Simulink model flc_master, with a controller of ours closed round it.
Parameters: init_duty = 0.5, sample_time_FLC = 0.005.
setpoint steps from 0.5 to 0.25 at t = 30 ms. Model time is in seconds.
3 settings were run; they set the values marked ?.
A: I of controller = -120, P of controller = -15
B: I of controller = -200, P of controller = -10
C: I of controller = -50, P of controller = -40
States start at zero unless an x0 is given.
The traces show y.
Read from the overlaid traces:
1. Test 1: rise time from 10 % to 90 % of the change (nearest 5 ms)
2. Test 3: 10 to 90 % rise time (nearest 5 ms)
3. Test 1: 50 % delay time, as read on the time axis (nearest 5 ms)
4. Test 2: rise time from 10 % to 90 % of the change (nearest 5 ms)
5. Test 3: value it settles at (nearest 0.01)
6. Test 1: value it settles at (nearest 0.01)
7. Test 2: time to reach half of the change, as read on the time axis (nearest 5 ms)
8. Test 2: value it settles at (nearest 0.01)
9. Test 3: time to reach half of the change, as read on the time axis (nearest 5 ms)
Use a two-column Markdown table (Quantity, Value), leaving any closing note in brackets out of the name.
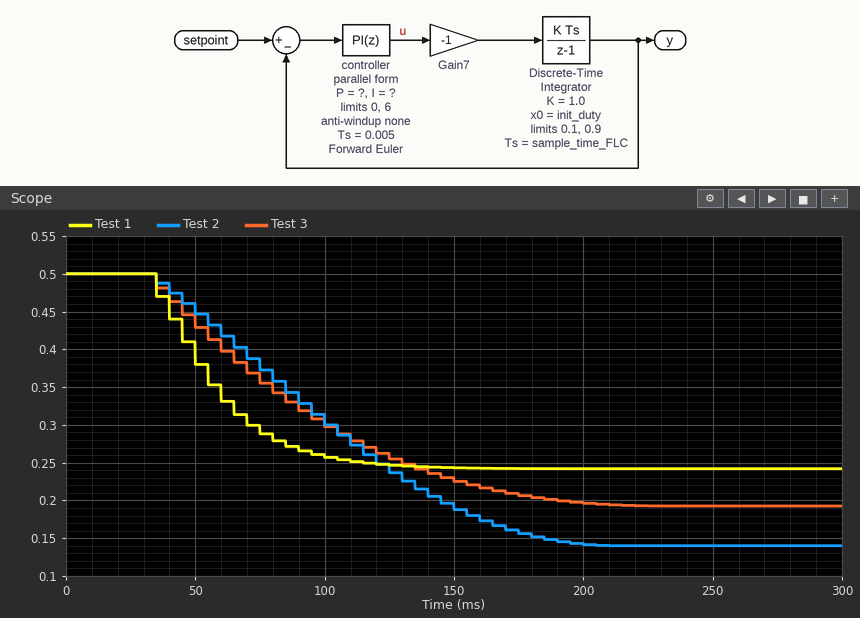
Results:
| Quantity | Value |
|---|---|
| Test 1: rise time from 10 % to 90 % of the change | 55 ms |
| Test 3: 10 to 90 % rise time | 115 ms |
| Test 1: 50 % delay time, as read on the time axis | 55 ms |
| Test 2: rise time from 10 % to 90 % of the change | 115 ms |
| Test 3: value it settles at | 0.19 |
| Test 1: value it settles at | 0.24 |
| Test 2: time to reach half of the change, as read on the time axis | 95 ms |
| Test 2: value it settles at | 0.14 |
| Test 3: time to reach half of the change, as read on the time axis | 80 ms |
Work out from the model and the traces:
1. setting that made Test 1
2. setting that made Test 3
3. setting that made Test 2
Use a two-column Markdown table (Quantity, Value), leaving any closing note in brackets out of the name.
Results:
| Quantity | Value |
|---|---|
| setting that made Test 1 | C |
| setting that made Test 3 | A |
| setting that made Test 2 | B |
